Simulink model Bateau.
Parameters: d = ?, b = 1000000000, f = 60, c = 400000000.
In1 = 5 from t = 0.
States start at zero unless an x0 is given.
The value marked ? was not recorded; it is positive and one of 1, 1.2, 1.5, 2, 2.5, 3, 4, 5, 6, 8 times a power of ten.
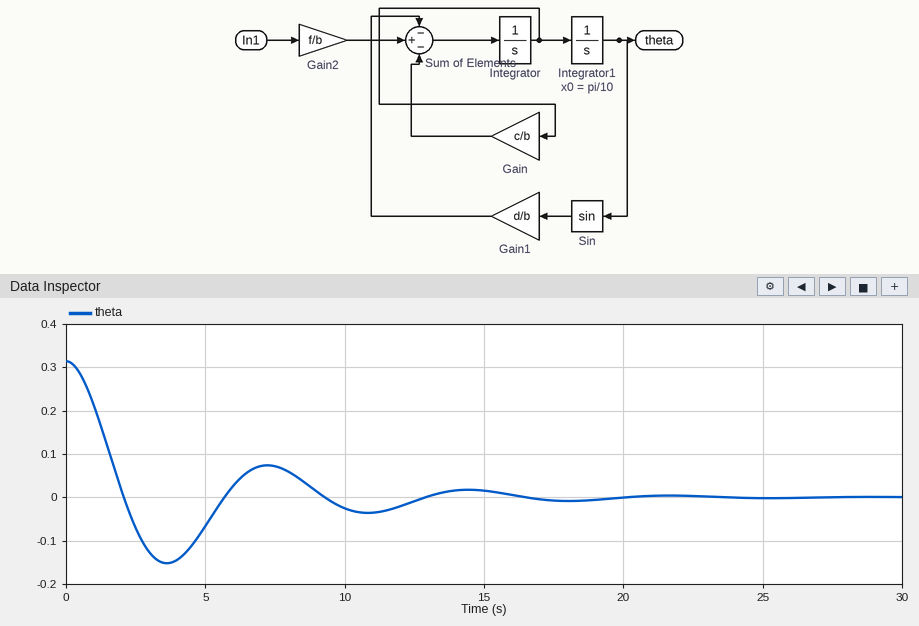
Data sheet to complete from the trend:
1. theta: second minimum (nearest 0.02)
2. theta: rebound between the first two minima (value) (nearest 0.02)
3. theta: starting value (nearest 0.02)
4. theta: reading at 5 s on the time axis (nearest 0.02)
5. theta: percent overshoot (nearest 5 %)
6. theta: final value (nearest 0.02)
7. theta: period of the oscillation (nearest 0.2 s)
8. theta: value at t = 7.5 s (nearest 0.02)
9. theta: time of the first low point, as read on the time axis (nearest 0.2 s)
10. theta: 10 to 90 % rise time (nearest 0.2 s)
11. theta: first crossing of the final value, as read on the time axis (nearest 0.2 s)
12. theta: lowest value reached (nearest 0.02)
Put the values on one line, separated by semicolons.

-0.04; 0.08; 0.32; -0.06; 50 %; 0.00; 7.2 s; 0.08; 3.6 s; 1.4 s; 2.0 s; -0.16
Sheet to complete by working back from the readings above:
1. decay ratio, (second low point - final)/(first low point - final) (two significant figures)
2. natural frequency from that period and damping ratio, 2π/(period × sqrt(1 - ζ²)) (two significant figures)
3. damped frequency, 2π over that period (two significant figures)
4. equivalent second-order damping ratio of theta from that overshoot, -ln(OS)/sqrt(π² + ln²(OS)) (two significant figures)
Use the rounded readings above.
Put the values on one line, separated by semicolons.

0.25; 0.89 rad/s; 0.87 rad/s; 0.22
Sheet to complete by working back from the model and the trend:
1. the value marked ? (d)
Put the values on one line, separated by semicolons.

8e+08
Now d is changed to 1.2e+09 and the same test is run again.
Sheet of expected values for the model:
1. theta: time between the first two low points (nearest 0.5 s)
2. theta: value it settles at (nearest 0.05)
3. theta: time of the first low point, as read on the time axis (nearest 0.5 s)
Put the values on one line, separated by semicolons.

6.0 s; 0.00; 3.0 s
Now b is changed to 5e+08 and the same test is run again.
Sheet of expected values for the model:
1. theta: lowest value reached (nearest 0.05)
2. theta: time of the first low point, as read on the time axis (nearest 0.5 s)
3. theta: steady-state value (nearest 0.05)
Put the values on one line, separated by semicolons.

-0.10; 2.5 s; 0.00
